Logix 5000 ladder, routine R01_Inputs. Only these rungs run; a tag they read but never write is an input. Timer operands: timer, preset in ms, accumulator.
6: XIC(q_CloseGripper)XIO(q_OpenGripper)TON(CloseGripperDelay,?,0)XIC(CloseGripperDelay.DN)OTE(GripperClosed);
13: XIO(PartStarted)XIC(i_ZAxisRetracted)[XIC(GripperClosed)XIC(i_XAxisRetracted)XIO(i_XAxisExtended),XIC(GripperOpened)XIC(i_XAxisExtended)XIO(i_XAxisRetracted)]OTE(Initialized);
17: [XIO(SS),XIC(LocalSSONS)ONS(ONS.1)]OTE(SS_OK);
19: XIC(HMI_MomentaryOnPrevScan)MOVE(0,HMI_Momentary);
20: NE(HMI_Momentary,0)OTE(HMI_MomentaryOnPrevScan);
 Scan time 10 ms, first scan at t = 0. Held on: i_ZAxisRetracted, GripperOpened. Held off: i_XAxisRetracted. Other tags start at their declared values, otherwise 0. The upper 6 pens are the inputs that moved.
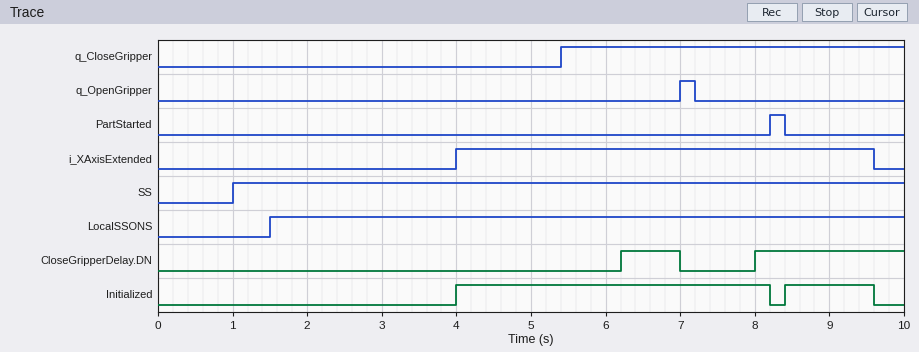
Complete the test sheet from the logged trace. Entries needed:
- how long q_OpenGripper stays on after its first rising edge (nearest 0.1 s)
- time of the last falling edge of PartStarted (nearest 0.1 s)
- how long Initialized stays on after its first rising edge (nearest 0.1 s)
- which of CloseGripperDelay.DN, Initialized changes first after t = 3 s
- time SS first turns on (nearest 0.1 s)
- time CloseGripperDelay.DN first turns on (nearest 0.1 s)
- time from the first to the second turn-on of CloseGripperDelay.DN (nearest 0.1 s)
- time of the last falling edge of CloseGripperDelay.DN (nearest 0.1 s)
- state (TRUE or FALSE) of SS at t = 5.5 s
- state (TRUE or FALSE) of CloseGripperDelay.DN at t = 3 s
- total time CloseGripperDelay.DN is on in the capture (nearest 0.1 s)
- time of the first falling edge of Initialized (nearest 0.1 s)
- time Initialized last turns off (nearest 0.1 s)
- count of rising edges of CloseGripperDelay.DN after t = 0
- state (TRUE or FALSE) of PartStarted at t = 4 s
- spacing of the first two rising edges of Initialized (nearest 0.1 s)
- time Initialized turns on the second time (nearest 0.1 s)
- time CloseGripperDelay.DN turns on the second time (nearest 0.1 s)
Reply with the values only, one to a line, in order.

0.2 s
8.4 s
4.2 s
Initialized
1.0 s
6.2 s
1.8 s
7.0 s
TRUE
FALSE
2.8 s
8.2 s
9.6 s
2
FALSE
4.4 s
8.4 s
8.0 s
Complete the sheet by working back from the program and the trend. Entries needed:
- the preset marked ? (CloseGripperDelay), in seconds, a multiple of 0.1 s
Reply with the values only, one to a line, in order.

0.8 s
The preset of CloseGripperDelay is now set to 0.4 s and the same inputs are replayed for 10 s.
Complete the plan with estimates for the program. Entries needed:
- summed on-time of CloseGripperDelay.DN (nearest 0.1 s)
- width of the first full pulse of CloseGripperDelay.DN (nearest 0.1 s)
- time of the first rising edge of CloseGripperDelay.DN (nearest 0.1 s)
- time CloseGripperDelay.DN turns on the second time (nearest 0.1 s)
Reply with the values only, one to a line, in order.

3.6 s
1.2 s
5.8 s
7.6 s
